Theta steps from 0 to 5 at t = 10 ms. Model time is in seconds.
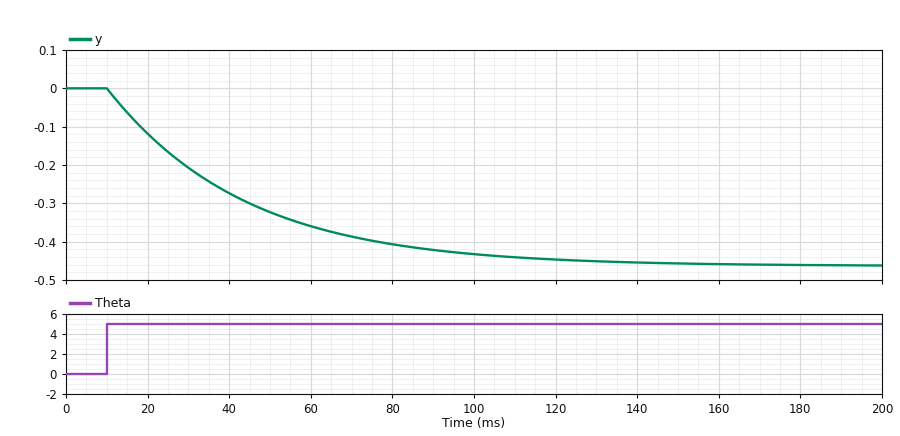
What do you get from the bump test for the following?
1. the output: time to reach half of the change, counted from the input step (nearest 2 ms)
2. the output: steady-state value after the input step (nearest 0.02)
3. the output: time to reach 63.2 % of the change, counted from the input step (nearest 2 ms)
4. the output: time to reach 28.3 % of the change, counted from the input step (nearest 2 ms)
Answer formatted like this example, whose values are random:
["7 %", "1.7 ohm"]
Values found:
["24 ms", "-0.46", "34 ms", "12 ms"]
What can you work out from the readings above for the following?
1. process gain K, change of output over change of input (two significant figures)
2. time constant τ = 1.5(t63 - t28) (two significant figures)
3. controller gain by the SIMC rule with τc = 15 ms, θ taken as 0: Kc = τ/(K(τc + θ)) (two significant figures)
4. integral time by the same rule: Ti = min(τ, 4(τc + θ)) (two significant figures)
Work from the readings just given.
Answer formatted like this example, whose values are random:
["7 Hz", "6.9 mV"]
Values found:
["-0.092", "33 ms", "-24", "33 ms"]
